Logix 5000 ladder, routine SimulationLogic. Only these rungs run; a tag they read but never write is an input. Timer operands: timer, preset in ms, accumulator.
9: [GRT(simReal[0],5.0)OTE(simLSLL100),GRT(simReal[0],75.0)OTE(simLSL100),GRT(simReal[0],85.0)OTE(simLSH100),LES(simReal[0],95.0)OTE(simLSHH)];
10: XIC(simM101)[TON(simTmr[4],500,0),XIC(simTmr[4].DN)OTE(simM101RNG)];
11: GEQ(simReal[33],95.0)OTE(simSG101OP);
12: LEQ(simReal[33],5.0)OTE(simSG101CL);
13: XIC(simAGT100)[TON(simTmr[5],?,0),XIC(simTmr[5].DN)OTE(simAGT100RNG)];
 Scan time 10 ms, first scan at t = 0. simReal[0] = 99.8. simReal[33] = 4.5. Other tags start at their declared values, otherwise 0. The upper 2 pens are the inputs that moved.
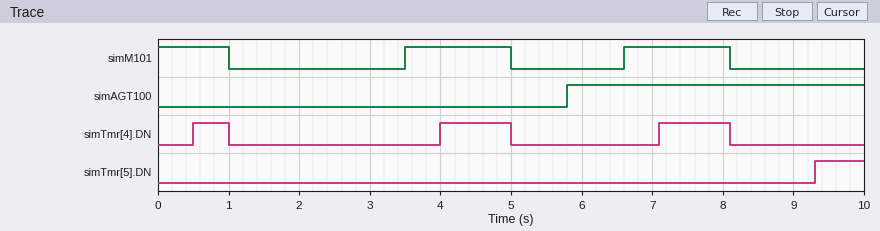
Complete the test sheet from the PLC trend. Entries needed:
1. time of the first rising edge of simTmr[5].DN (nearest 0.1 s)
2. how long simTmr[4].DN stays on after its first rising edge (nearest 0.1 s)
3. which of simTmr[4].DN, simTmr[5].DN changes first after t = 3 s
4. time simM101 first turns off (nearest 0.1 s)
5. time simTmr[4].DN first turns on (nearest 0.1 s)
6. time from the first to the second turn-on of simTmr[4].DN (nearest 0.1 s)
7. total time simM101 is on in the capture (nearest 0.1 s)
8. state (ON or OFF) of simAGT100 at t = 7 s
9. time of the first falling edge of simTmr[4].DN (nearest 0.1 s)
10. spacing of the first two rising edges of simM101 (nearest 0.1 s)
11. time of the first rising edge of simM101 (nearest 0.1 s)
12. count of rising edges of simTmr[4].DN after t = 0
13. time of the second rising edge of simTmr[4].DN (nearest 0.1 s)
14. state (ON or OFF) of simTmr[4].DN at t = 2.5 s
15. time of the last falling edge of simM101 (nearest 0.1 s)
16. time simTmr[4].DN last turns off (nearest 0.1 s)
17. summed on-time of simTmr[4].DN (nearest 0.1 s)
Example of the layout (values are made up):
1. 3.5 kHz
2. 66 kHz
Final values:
1. 9.3 s
2. 0.5 s
3. simTmr[4].DN
4. 1.0 s
5. 0.5 s
6. 3.5 s
7. 4.0 s
8. ON
9. 1.0 s
10. 3.1 s
11. 3.5 s
12. 3
13. 4.0 s
14. OFF
15. 8.1 s
16. 8.1 s
17. 2.5 s
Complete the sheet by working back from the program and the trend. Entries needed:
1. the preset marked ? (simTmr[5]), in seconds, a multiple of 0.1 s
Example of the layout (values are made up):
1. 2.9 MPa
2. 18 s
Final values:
1. 3.5 s
